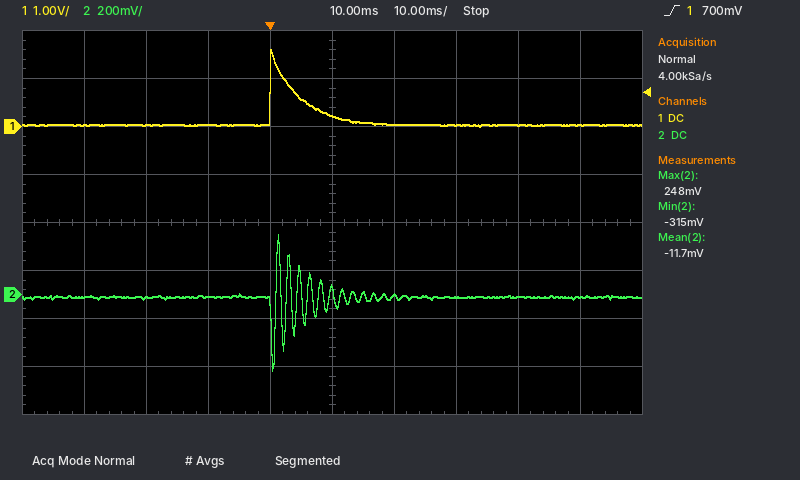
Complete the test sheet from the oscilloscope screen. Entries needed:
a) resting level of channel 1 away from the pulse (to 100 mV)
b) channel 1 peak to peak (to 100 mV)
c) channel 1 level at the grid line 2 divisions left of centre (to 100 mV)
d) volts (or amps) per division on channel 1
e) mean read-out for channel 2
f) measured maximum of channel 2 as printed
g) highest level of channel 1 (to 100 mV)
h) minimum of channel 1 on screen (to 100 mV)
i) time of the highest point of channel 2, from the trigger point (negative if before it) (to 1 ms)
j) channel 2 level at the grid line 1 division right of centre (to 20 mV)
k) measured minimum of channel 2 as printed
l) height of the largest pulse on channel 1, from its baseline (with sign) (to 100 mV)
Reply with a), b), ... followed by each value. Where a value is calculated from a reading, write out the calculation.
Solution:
a) 0.0 V
b) 1.6 V − (0.0 V) = 1.6 V
c) 0.0 V
d) 1 V
e) -11.7 mV
f) 248 mV
g) 1.6 V
h) 0.0 V
i) +1 ms
j) 0 mV
k) -315 mV
l) 1.6 V − (0.0 V) = +1.6 V
